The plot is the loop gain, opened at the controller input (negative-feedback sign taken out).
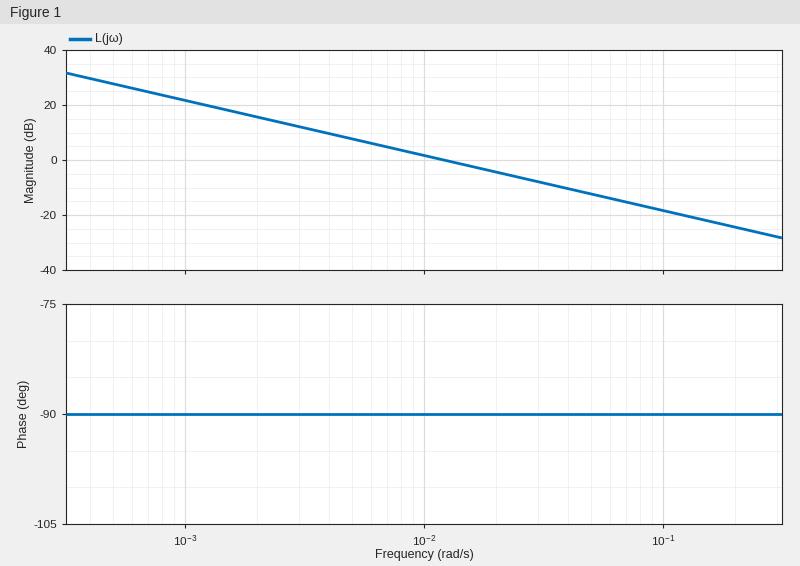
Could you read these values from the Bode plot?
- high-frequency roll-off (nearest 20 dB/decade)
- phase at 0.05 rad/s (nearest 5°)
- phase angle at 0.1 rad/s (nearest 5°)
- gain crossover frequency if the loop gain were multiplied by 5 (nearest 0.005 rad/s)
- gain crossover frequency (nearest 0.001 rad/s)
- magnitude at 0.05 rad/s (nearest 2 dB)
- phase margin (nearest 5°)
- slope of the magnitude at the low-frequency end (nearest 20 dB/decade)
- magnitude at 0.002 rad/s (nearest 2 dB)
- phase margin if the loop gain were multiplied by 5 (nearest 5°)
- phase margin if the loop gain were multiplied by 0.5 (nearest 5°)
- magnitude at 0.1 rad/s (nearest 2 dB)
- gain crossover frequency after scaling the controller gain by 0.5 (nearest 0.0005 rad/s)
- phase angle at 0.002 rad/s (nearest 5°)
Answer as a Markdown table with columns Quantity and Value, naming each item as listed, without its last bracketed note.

| Quantity | Value |
|---|---|
| high-frequency roll-off | -20 dB/decade |
| phase at 0.05 rad/s | -90° |
| phase angle at 0.1 rad/s | -90° |
| gain crossover frequency if the loop gain were multiplied by 5 | 0.060 rad/s |
| gain crossover frequency | 0.012 rad/s |
| magnitude at 0.05 rad/s | -12 dB |
| phase margin | 90° |
| slope of the magnitude at the low-frequency end | -20 dB/decade |
| magnitude at 0.002 rad/s | 16 dB |
| phase margin if the loop gain were multiplied by 5 | 90° |
| phase margin if the loop gain were multiplied by 0.5 | 90° |
| magnitude at 0.1 rad/s | -18 dB |
| gain crossover frequency after scaling the controller gain by 0.5 | 0.0060 rad/s |
| phase angle at 0.002 rad/s | -90° |
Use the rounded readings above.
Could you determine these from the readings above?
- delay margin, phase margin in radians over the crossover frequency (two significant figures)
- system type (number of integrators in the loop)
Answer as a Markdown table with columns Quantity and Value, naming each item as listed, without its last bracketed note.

| Quantity | Value |
|---|---|
| delay margin, phase margin in radians over the crossover frequency | 130 s |
| system type | 1 |
